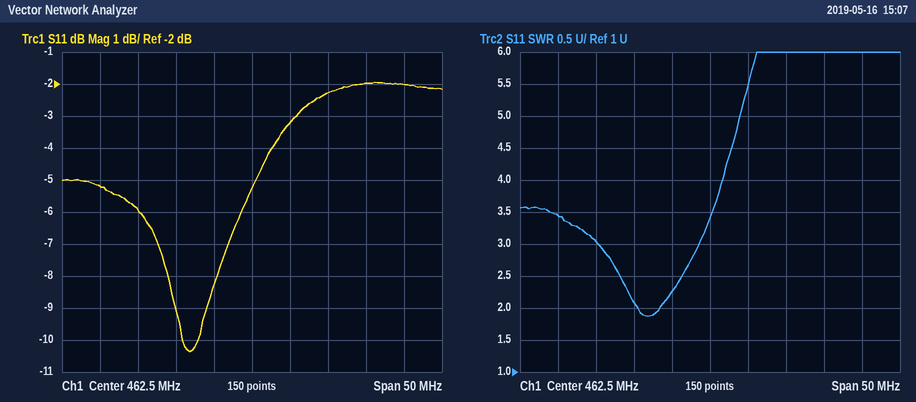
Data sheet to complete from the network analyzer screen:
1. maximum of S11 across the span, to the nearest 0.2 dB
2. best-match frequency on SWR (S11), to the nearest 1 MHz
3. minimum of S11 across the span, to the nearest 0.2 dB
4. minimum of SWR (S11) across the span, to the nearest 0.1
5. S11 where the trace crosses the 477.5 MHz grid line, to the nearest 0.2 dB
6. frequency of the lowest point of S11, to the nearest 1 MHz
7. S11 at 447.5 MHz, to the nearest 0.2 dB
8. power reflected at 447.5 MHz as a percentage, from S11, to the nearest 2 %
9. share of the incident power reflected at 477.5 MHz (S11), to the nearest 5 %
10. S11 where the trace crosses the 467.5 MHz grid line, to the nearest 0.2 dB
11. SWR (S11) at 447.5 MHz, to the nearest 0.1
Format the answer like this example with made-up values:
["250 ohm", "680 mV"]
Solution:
["-2.0 dB", "454 MHz", "-10.4 dB", "1.9", "-2.0 dB", "454 MHz", "-6.0 dB", "26 %", "65 %", "-3.2 dB", "3.0"]
